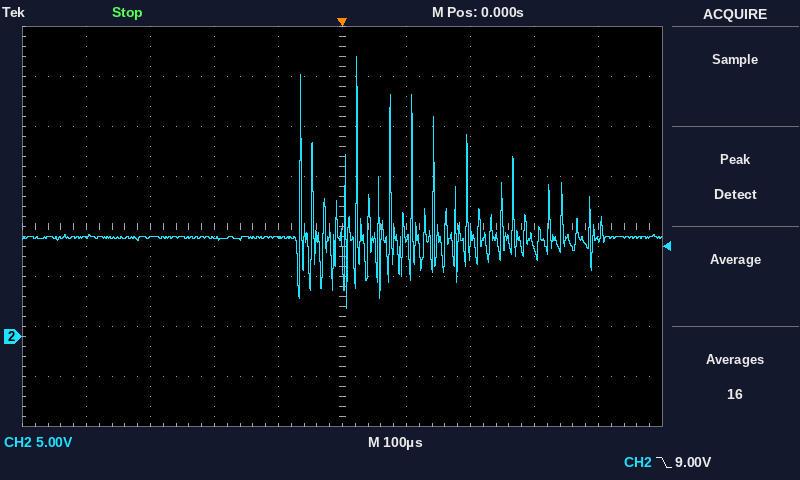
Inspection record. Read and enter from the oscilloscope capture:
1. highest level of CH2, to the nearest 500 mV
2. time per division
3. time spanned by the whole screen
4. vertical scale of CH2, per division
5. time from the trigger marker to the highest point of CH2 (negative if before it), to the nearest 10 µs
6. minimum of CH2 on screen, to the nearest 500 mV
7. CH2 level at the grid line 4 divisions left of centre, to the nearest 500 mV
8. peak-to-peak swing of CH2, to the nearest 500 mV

28.0 V
100 µs
1 ms
5 V
+20 µs
3.0 V
10.0 V
25.0 V
